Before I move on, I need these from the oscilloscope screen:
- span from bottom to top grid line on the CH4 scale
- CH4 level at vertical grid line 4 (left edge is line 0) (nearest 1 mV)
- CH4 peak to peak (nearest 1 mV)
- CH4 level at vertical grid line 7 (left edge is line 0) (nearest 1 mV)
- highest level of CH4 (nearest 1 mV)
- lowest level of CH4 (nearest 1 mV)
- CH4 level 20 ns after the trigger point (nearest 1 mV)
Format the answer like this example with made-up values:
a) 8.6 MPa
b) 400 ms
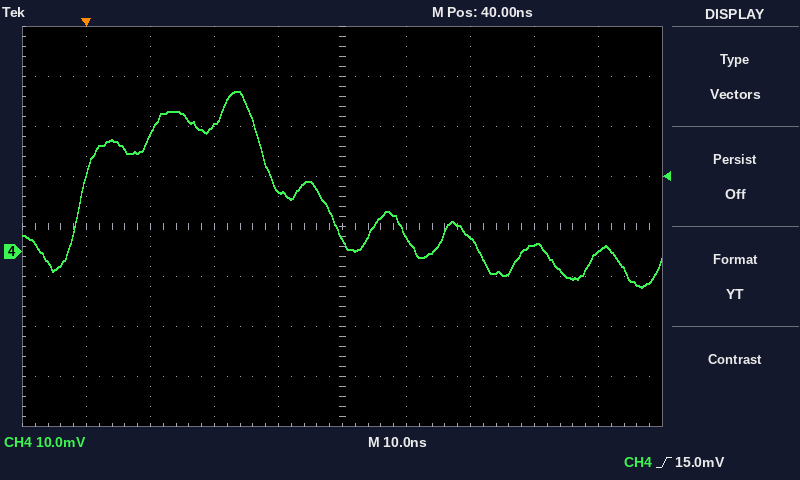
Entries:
a) 80 mV
b) 12 mV
c) 39 mV
d) 3 mV
e) 32 mV
f) -7 mV
g) 25 mV
